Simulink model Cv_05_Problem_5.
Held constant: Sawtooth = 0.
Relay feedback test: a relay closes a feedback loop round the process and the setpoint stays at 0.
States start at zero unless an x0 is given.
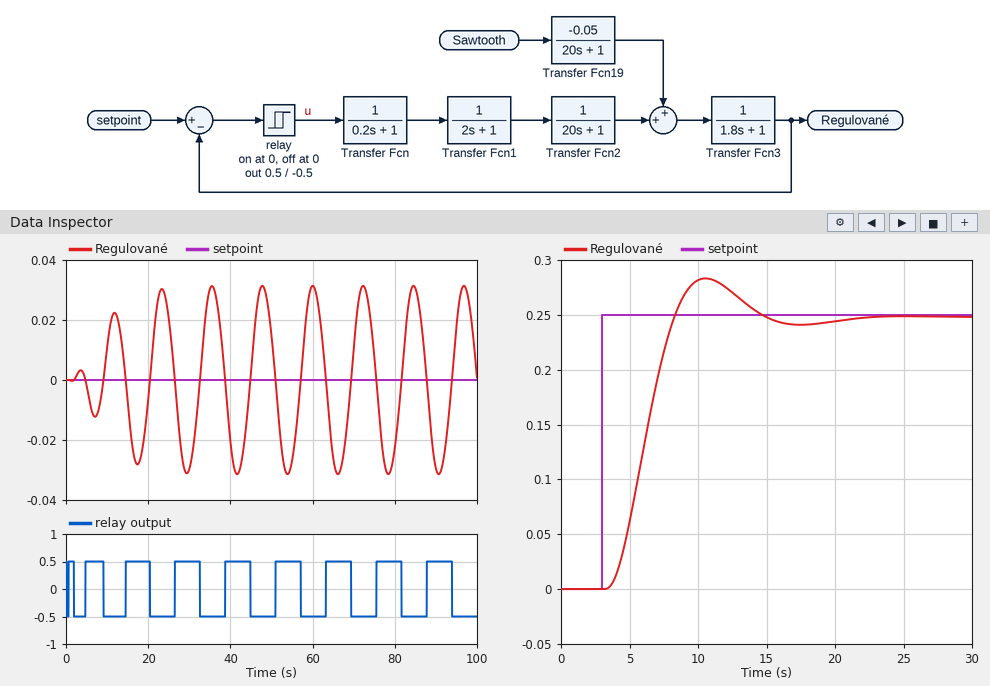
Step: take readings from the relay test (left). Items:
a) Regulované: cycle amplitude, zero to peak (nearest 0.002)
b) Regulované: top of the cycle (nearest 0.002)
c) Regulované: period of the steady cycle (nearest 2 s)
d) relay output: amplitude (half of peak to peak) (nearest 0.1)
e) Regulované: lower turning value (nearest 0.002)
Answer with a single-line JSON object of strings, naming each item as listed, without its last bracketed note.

{"Regulované: cycle amplitude, zero to peak": "0.032", "Regulované: top of the cycle": "0.032", "Regulované: period of the steady cycle": "12 s", "relay output: amplitude (half of peak to peak)": "0.5", "Regulované: lower turning value": "-0.032"}
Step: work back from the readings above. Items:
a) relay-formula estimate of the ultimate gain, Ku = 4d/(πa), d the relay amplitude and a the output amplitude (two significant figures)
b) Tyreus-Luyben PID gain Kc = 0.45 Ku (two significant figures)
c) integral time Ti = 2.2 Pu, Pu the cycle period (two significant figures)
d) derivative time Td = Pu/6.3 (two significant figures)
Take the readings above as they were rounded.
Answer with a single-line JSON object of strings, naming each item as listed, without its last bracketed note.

{"relay-formula estimate of the ultimate gain, Ku = 4d/(πa), d the relay amplitude and a the output amplitude": "20", "Tyreus-Luyben PID gain Kc = 0.45 Ku": "9.0", "integral time Ti = 2.2 Pu, Pu the cycle period": "26 s", "derivative time Td = Pu/6.3": "1.9 s"}
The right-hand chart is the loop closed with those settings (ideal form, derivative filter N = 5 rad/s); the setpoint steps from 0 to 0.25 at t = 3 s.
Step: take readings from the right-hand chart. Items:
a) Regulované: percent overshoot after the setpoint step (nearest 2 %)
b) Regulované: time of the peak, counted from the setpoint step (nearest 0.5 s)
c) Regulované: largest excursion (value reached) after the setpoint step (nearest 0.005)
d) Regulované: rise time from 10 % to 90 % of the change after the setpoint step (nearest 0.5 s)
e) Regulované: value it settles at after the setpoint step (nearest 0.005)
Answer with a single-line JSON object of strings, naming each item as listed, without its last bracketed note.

{"Regulované: percent overshoot after the setpoint step": "14 %", "Regulované: time of the peak, counted from the setpoint step": "7.5 s", "Regulované: largest excursion (value reached) after the setpoint step": "0.285", "Regulované: rise time from 10 % to 90 % of the change after the setpoint step": "3.5 s", "Regulované: value it settles at after the setpoint step": "0.250"}
